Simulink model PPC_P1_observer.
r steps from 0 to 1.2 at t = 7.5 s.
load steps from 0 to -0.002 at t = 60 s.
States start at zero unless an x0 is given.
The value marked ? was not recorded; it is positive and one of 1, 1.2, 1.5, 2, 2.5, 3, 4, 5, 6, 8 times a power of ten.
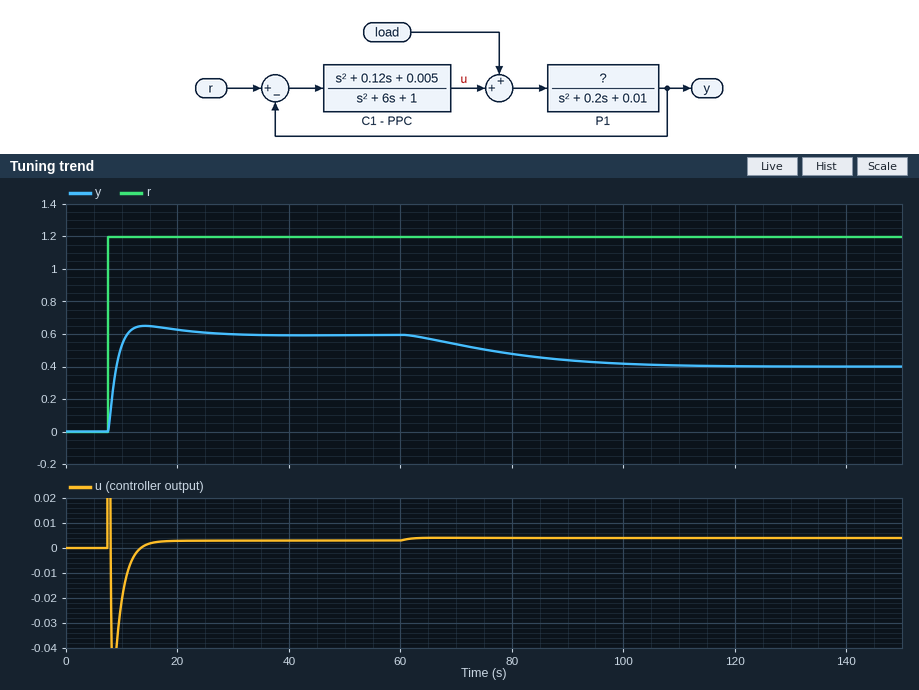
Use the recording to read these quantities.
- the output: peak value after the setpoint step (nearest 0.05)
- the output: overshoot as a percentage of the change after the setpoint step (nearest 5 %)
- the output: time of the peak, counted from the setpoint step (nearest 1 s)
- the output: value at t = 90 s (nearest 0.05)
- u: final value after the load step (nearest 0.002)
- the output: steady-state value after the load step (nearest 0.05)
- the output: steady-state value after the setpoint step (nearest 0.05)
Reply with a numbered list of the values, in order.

1. 0.65
2. 10 %
3. 7 s
4. 0.45
5. 0.004
6. 0.40
7. 0.60
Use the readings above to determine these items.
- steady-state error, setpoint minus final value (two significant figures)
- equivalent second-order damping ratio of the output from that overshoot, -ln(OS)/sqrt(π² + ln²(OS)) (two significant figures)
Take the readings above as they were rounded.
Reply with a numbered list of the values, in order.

1. 0.60
2. 0.59
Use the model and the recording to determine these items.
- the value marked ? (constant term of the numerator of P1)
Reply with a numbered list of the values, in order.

1. 2
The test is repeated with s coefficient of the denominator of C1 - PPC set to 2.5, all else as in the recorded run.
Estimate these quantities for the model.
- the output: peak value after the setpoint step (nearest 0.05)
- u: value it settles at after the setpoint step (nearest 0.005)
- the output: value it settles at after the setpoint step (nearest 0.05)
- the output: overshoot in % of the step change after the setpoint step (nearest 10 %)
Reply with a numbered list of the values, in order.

1. 0.75
2. 0.005
3. 0.60
4. 30 %
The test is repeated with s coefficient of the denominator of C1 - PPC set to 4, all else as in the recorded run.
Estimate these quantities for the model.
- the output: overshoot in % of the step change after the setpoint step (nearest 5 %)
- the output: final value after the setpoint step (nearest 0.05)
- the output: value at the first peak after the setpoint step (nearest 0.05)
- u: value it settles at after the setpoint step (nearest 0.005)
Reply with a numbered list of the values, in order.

1. 15 %
2. 0.60
3. 0.70
4. 0.005
